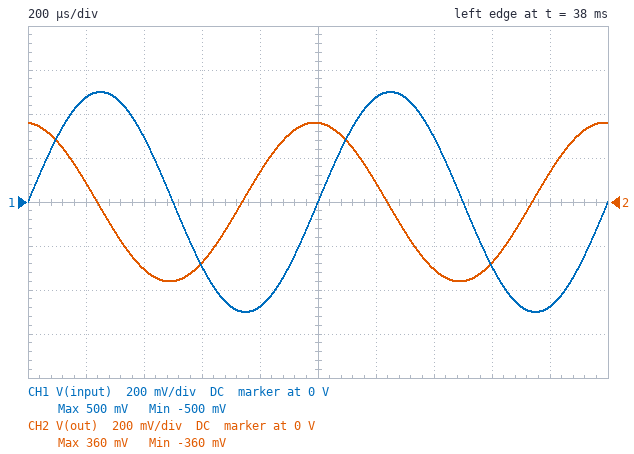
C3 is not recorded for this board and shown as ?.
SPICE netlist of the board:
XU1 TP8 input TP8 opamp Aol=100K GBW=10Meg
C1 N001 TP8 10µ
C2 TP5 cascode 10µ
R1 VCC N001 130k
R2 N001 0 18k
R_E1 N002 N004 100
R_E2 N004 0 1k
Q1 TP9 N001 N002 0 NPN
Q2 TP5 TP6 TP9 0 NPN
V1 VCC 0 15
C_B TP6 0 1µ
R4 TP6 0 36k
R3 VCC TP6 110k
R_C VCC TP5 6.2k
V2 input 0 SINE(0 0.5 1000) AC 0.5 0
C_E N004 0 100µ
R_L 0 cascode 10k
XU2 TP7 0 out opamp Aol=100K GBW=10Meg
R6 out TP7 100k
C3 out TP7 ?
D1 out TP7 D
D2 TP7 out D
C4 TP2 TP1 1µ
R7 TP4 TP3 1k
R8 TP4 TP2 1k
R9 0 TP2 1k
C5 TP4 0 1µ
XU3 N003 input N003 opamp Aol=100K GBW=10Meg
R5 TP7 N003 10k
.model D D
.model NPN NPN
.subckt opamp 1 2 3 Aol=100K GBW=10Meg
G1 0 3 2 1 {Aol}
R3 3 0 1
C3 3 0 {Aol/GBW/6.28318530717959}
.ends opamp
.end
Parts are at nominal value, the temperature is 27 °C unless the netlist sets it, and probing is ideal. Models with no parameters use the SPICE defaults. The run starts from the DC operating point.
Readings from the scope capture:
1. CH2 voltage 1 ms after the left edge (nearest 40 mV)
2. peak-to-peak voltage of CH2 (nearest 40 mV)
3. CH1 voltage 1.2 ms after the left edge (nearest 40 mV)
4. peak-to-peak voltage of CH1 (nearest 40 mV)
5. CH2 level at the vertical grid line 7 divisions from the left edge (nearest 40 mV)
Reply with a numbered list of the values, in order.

1. 360 mV
2. 720 mV
3. 480 mV
4. 1.00 V
5. -320 mV
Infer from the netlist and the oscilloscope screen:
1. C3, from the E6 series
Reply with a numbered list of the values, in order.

1. 22 nF
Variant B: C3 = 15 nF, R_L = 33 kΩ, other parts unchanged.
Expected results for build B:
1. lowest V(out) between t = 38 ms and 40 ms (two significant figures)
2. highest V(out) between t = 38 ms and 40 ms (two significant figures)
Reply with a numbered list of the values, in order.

1. -520 mV
2. 520 mV
